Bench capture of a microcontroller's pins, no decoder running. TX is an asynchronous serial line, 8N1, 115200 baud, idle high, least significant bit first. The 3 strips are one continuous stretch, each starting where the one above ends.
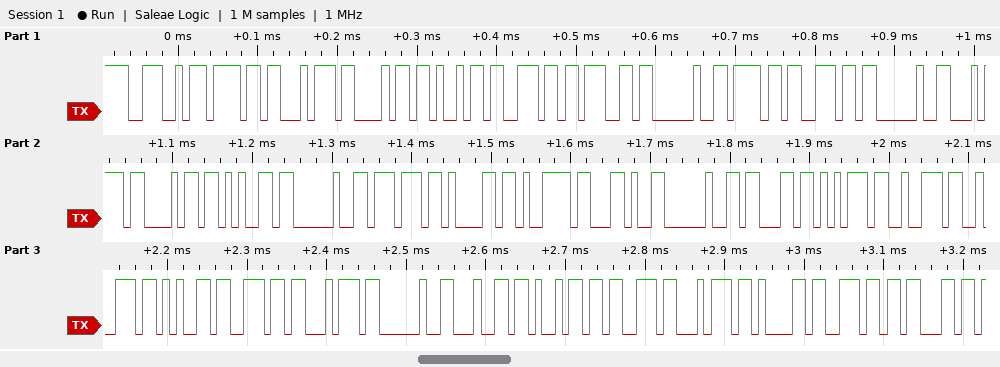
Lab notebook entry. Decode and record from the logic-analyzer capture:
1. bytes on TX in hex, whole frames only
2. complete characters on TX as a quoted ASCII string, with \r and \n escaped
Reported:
4E 6F 74 68 69 6E 67 20 6F 6E 20 74 68 65 20 77 61 79 2C 20 63 75 72 72 65 6E 74 20 64 69 73 74 61 6E 63
"Nothing on the way, current distanc"
